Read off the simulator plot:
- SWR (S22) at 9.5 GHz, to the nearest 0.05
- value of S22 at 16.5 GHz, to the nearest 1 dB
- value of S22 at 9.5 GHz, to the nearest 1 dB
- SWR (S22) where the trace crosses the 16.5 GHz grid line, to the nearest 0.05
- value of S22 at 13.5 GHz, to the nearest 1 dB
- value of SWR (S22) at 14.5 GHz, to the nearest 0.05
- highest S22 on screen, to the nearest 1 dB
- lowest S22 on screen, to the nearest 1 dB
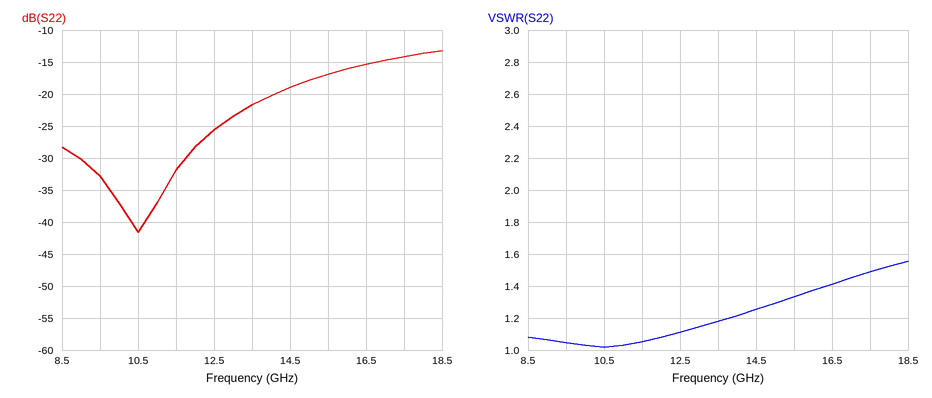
1.05
-15 dB
-33 dB
1.40
-22 dB
1.25
-13 dB
-42 dB
